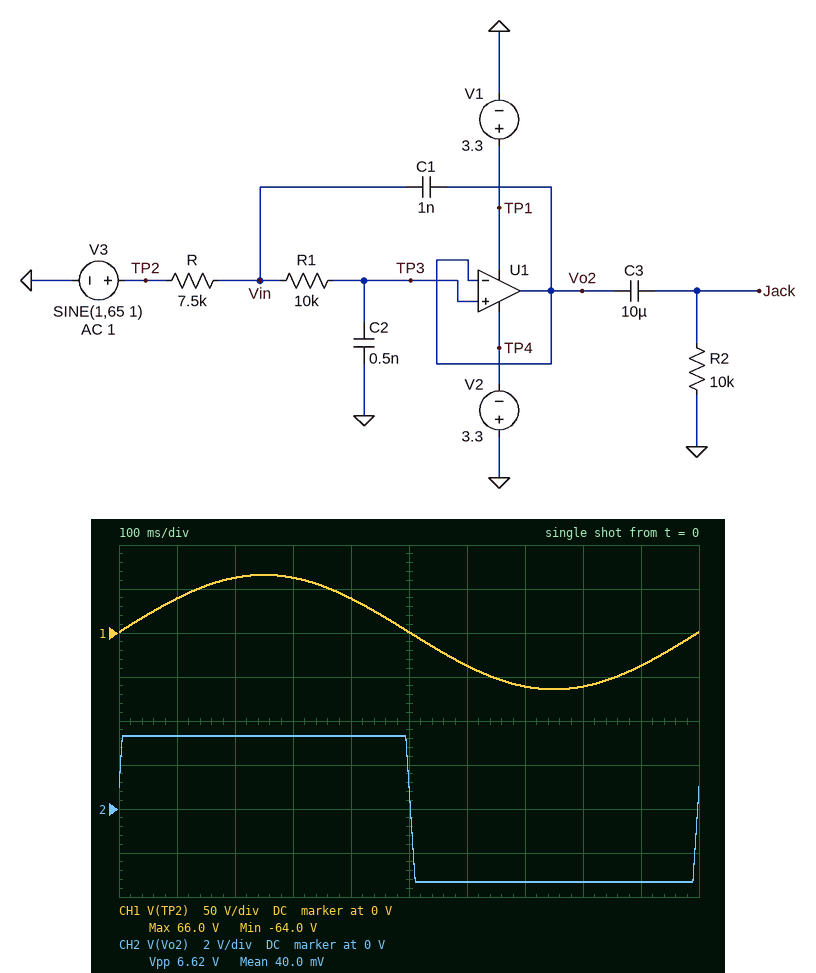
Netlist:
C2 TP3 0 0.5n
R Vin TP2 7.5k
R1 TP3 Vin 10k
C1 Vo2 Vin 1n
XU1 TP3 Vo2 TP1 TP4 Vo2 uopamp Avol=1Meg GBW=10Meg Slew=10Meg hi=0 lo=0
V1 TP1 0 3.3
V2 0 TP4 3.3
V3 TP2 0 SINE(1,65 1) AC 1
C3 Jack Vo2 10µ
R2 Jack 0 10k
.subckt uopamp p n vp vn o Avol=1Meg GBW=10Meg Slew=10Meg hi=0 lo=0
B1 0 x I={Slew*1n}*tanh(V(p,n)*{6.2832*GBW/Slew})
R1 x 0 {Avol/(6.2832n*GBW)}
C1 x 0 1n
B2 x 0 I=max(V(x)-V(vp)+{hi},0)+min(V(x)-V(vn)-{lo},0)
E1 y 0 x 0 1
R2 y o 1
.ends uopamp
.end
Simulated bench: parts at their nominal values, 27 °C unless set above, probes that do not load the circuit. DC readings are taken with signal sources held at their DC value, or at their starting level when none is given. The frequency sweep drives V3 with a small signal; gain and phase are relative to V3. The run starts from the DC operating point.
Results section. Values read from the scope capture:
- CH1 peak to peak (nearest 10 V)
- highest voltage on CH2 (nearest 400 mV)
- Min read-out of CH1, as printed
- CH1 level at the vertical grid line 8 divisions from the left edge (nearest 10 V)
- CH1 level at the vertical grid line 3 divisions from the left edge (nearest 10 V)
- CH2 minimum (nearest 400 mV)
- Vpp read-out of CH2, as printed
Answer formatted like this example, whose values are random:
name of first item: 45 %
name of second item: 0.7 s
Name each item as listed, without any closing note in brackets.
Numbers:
CH1 peak to peak: 130 V
highest voltage on CH2: 3.2 V
Min read-out of CH1, as printed: -64.0 V
CH1 level at the vertical grid line 8 divisions from the left edge: -60 V
CH1 level at the vertical grid line 3 divisions from the left edge: 60 V
CH2 minimum: -3.2 V
Vpp read-out of CH2, as printed: 6.62 V
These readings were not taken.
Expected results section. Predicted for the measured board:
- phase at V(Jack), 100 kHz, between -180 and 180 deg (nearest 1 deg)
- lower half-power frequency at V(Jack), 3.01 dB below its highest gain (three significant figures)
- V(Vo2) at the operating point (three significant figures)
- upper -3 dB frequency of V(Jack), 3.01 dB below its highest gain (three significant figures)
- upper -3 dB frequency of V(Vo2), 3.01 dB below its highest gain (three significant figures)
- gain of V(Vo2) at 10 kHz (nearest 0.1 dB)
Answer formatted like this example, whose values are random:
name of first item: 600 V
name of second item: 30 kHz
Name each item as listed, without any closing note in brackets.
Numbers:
phase at V(Jack), 100 kHz, between -180 and 180 deg: -159 deg
lower half-power frequency at V(Jack), 3.01 dB below its highest gain: 1.59 Hz
V(Vo2) at the operating point: 1.00 V
upper -3 dB frequency of V(Jack), 3.01 dB below its highest gain: 25.7 kHz
upper -3 dB frequency of V(Vo2), 3.01 dB below its highest gain: 25.7 kHz
gain of V(Vo2) at 10 kHz: -0.1 dB
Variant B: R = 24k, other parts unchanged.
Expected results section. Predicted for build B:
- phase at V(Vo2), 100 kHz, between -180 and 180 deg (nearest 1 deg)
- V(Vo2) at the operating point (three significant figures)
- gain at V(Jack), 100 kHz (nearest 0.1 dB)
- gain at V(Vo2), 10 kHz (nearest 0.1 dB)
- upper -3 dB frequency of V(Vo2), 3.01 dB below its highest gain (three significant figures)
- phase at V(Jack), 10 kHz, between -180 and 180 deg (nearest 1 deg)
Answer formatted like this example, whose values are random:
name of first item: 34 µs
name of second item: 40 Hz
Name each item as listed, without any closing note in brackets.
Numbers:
phase at V(Vo2), 100 kHz, between -180 and 180 deg: -168 deg
V(Vo2) at the operating point: 1.00 V
gain at V(Jack), 100 kHz: -33.6 dB
gain at V(Vo2), 10 kHz: -1.5 dB
upper -3 dB frequency of V(Vo2), 3.01 dB below its highest gain: 13.1 kHz
phase at V(Jack), 10 kHz, between -180 and 180 deg: -64 deg
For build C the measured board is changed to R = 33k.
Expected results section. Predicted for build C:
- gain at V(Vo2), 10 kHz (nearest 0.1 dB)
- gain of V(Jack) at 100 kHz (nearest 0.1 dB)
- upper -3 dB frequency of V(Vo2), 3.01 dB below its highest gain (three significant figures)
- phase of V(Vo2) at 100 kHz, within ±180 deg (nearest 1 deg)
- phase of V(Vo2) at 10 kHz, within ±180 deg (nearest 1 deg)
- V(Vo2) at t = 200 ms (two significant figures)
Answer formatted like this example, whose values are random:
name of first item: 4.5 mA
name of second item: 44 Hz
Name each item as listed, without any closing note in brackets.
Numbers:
gain at V(Vo2), 10 kHz: -2.9 dB
gain of V(Jack) at 100 kHz: -36.4 dB
upper -3 dB frequency of V(Vo2), 3.01 dB below its highest gain: 10.2 kHz
phase of V(Vo2) at 100 kHz, within ±180 deg: -169 deg
phase of V(Vo2) at 10 kHz, within ±180 deg: -76 deg
V(Vo2) at t = 200 ms: 3.3 V
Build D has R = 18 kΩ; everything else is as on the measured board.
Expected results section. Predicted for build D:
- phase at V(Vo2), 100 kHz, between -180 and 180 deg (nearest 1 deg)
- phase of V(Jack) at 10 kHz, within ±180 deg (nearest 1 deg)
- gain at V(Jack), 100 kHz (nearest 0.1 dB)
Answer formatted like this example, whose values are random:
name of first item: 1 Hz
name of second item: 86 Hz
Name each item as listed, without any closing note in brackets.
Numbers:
phase at V(Vo2), 100 kHz, between -180 and 180 deg: -166 deg
phase of V(Jack) at 10 kHz, within ±180 deg: -54 deg
gain at V(Jack), 100 kHz: -31.1 dB
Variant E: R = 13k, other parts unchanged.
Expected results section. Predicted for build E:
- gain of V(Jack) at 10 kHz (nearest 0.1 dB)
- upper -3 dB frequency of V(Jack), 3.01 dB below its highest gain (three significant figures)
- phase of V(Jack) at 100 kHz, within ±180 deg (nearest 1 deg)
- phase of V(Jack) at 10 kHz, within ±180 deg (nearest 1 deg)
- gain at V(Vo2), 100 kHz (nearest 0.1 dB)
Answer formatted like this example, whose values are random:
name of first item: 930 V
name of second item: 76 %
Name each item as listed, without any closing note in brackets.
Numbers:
gain of V(Jack) at 10 kHz: -0.3 dB
upper -3 dB frequency of V(Jack), 3.01 dB below its highest gain: 19.6 kHz
phase of V(Jack) at 100 kHz, within ±180 deg: -164 deg
phase of V(Jack) at 10 kHz, within ±180 deg: -44 deg
gain at V(Vo2), 100 kHz: -28.2 dB
